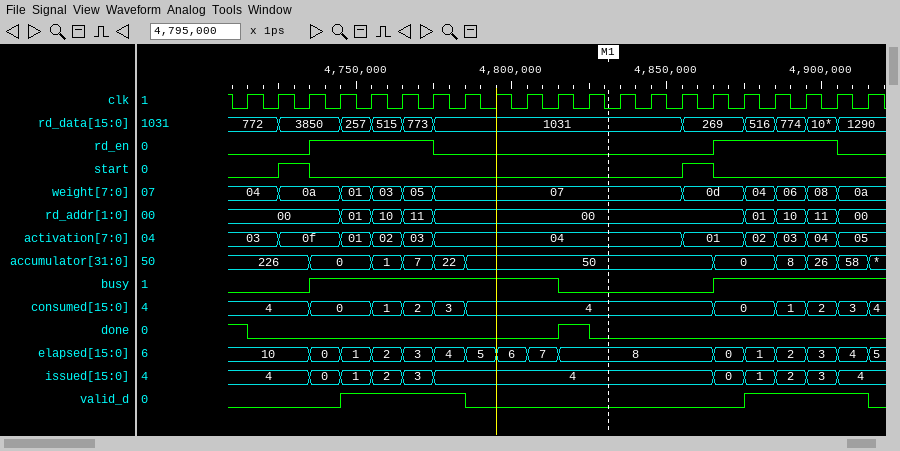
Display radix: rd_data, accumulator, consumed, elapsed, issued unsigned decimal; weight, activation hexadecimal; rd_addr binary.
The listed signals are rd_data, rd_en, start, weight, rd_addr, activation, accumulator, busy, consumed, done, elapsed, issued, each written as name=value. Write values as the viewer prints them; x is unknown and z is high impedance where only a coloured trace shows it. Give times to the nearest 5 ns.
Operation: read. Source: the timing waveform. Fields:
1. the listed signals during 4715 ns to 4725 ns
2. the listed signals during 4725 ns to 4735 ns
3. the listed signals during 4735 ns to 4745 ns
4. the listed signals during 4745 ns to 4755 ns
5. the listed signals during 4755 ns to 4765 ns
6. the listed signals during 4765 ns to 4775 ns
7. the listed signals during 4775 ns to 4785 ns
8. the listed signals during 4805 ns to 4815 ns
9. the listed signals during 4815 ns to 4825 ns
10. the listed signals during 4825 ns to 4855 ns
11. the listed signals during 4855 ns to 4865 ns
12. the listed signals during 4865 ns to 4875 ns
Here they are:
rd_data=772, rd_en=0, start=0, weight=04, rd_addr=00, activation=03, accumulator=226, busy=0, consumed=4, done=0, elapsed=10, issued=4
rd_data=3850, rd_en=0, start=1, weight=0a, rd_addr=00, activation=0f, accumulator=226, busy=0, consumed=4, done=0, elapsed=10, issued=4
rd_data=3850, rd_en=1, start=0, weight=0a, rd_addr=00, activation=0f, accumulator=0, busy=1, consumed=0, done=0, elapsed=0, issued=0
rd_data=257, rd_en=1, start=0, weight=01, rd_addr=01, activation=01, accumulator=0, busy=1, consumed=0, done=0, elapsed=1, issued=1
rd_data=515, rd_en=1, start=0, weight=03, rd_addr=10, activation=02, accumulator=1, busy=1, consumed=1, done=0, elapsed=2, issued=2
rd_data=773, rd_en=1, start=0, weight=05, rd_addr=11, activation=03, accumulator=7, busy=1, consumed=2, done=0, elapsed=3, issued=3
rd_data=1031, rd_en=0, start=0, weight=07, rd_addr=00, activation=04, accumulator=22, busy=1, consumed=3, done=0, elapsed=4, issued=4
rd_data=1031, rd_en=0, start=0, weight=07, rd_addr=00, activation=04, accumulator=50, busy=1, consumed=4, done=0, elapsed=7, issued=4
rd_data=1031, rd_en=0, start=0, weight=07, rd_addr=00, activation=04, accumulator=50, busy=0, consumed=4, done=1, elapsed=8, issued=4
rd_data=1031, rd_en=0, start=0, weight=07, rd_addr=00, activation=04, accumulator=50, busy=0, consumed=4, done=0, elapsed=8, issued=4
rd_data=269, rd_en=0, start=1, weight=0d, rd_addr=00, activation=01, accumulator=50, busy=0, consumed=4, done=0, elapsed=8, issued=4
rd_data=269, rd_en=1, start=0, weight=0d, rd_addr=00, activation=01, accumulator=0, busy=1, consumed=0, done=0, elapsed=0, issued=0
